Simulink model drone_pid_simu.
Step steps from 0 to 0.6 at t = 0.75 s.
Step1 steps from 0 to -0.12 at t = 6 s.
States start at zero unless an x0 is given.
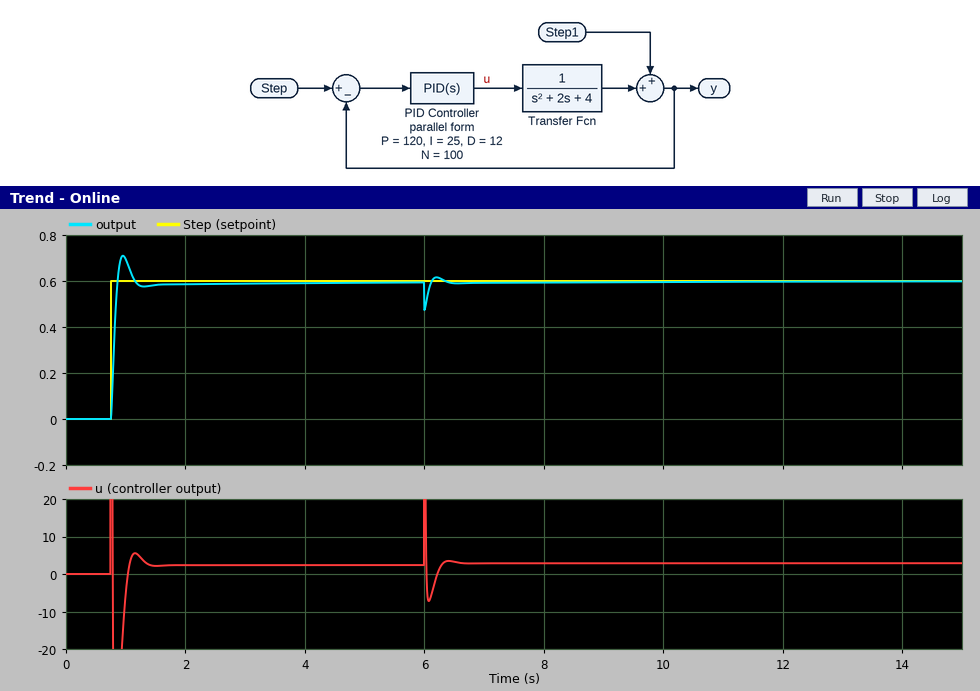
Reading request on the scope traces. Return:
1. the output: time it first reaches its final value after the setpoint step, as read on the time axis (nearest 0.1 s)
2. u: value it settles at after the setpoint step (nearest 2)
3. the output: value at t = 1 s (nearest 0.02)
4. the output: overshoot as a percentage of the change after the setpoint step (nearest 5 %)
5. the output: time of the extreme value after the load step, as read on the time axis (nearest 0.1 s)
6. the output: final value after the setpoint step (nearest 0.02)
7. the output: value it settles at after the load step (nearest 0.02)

0.9 s
2
0.70
20 %
6.0 s
0.60
0.60
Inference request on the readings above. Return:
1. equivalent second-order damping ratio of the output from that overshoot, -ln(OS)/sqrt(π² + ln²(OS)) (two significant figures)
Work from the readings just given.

0.46
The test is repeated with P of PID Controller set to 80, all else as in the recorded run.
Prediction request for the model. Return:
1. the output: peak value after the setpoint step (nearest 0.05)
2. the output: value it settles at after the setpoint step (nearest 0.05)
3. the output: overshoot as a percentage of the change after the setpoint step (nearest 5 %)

0.65
0.60
10 %
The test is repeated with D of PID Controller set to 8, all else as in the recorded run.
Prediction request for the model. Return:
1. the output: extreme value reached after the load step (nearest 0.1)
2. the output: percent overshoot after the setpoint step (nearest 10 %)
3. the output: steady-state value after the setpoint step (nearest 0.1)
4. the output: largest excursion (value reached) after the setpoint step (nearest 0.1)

0.5
30 %
0.6
0.8
